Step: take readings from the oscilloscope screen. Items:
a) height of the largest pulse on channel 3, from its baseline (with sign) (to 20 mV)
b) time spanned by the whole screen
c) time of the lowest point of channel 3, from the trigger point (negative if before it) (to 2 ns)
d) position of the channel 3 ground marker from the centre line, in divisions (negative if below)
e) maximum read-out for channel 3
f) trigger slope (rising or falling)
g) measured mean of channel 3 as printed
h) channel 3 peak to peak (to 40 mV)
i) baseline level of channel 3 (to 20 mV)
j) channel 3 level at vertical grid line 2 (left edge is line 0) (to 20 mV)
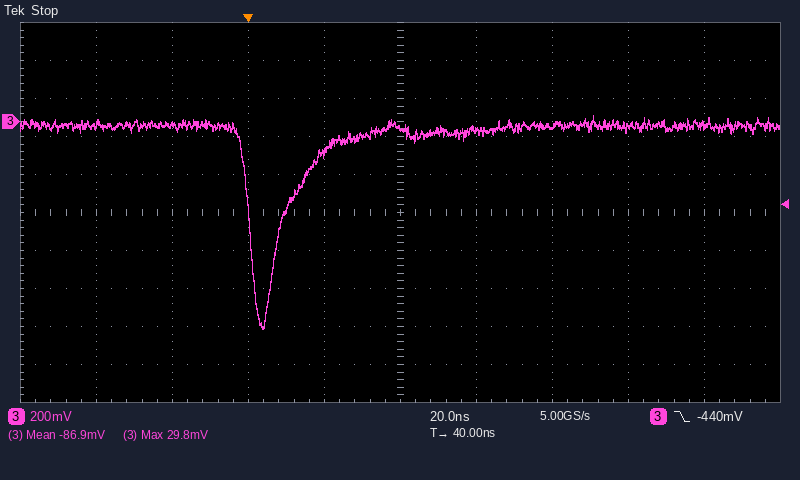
-1.06 V
200 ns
+4 ns
+2.4 div
29.8 mV
falling
-86.9 mV
1.12 V
-20 mV
-20 mV
